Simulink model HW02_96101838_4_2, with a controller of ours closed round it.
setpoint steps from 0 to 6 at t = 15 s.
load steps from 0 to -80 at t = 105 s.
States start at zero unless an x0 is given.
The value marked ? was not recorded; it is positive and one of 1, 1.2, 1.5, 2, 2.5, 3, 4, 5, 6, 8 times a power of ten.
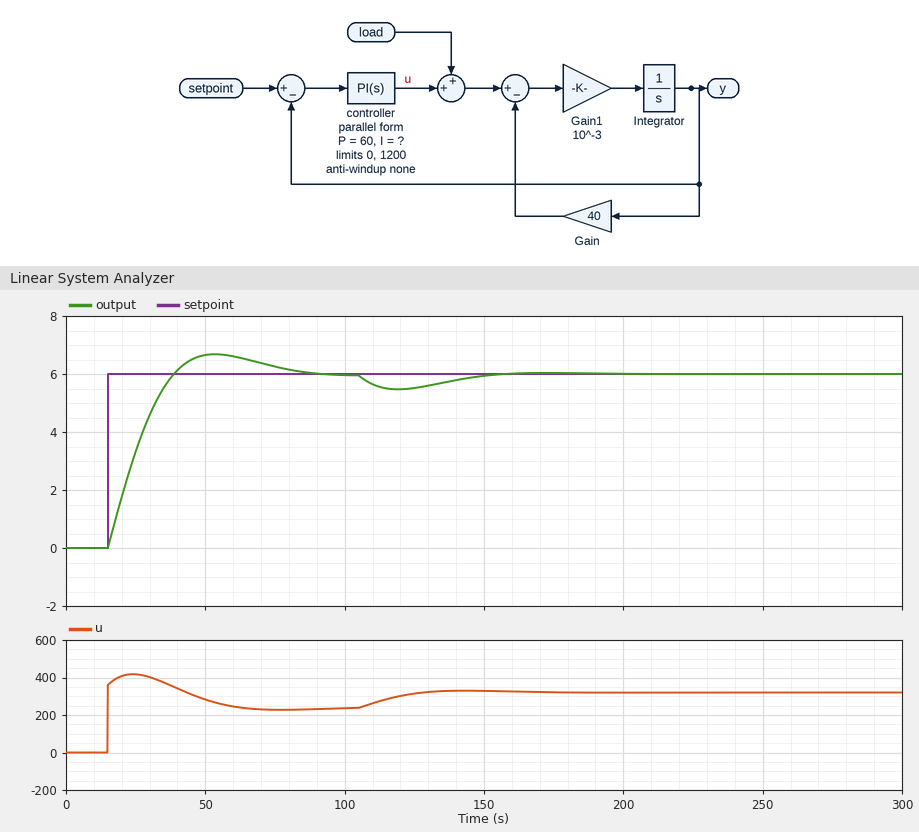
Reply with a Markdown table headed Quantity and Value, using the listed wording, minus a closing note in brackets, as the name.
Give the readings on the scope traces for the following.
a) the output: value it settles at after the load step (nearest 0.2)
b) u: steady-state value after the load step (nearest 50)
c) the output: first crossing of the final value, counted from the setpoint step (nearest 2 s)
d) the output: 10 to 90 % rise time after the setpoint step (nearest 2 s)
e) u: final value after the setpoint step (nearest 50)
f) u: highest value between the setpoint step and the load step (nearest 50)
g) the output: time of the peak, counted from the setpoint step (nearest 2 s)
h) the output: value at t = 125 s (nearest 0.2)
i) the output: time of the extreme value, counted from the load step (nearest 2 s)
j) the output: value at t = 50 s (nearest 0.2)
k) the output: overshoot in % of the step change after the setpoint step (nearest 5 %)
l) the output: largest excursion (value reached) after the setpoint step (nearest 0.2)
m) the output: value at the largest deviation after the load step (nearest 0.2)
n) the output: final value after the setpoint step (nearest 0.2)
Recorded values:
| Quantity | Value |
|---|---|
| the output: value it settles at after the load step | 6.0 |
| u: steady-state value after the load step | 300 |
| the output: first crossing of the final value, counted from the setpoint step | 24 s |
| the output: 10 to 90 % rise time after the setpoint step | 18 s |
| u: final value after the setpoint step | 250 |
| u: highest value between the setpoint step and the load step | 400 |
| the output: time of the peak, counted from the setpoint step | 38 s |
| the output: value at t = 125 s | 5.6 |
| the output: time of the extreme value, counted from the load step | 14 s |
| the output: value at t = 50 s | 6.6 |
| the output: overshoot in % of the step change after the setpoint step | 10 % |
| the output: largest excursion (value reached) after the setpoint step | 6.6 |
| the output: value at the largest deviation after the load step | 5.4 |
| the output: final value after the setpoint step | 6.0 |
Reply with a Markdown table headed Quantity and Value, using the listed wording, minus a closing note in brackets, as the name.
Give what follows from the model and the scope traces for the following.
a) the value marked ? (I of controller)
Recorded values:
| Quantity | Value |
|---|---|
| the value marked ? | 6 |
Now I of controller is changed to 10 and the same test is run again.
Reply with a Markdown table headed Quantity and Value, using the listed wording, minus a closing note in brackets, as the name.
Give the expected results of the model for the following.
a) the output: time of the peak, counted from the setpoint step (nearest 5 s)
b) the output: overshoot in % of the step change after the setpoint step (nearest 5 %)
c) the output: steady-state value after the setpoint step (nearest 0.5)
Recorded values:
| Quantity | Value |
|---|---|
| the output: time of the peak, counted from the setpoint step | 30 s |
| the output: overshoot in % of the step change after the setpoint step | 20 % |
| the output: steady-state value after the setpoint step | 6.0 |
